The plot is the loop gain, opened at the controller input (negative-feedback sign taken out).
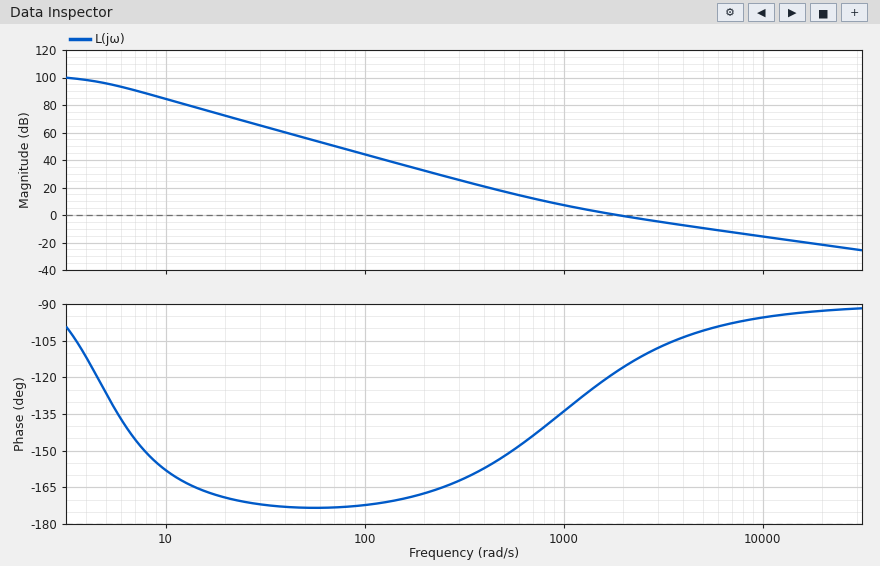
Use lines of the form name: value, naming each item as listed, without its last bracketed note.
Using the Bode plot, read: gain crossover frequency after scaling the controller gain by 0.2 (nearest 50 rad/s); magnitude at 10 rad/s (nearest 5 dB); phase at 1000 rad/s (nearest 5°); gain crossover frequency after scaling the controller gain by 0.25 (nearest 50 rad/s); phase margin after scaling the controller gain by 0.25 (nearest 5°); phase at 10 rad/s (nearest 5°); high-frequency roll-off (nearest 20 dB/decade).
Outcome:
gain crossover frequency after scaling the controller gain by 0.2: 600 rad/s
magnitude at 10 rad/s: 85 dB
phase at 1000 rad/s: -135°
gain crossover frequency after scaling the controller gain by 0.25: 700 rad/s
phase margin after scaling the controller gain by 0.25: 35°
phase at 10 rad/s: -160°
high-frequency roll-off: -20 dB/decade
